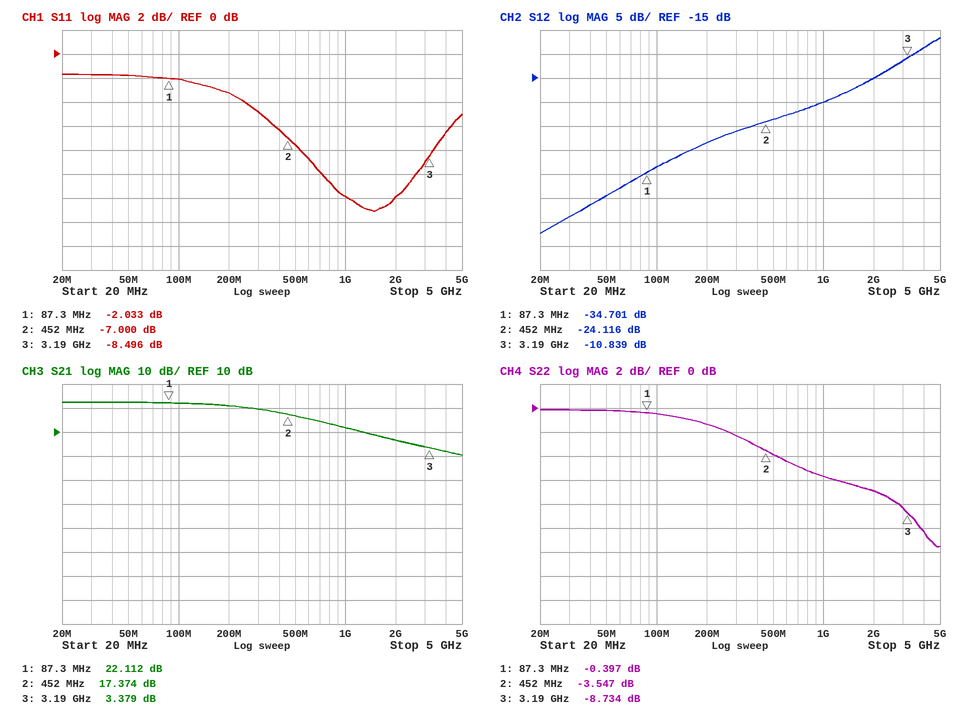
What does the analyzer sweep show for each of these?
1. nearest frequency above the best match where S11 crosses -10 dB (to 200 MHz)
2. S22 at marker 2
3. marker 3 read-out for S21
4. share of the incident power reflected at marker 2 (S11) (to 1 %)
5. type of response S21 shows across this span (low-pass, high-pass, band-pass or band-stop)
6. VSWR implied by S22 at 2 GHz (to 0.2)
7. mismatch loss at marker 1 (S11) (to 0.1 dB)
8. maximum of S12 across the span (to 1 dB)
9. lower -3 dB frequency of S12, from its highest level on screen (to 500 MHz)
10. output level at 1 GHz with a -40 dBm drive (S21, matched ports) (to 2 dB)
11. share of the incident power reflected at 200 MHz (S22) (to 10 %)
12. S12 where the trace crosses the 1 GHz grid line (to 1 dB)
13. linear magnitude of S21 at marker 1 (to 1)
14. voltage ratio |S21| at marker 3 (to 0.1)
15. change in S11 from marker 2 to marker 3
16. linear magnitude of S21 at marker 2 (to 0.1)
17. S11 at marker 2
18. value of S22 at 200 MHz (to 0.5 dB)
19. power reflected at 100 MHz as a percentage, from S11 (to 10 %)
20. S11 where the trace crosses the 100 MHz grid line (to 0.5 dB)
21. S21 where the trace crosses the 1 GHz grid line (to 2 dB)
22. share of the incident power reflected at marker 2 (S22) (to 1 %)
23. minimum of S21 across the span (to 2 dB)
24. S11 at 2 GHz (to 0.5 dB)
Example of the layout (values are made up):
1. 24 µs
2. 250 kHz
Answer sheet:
1. 2.6 GHz
2. -3.547 dB
3. 3.379 dB
4. 20 %
5. low-pass
6. 2.6
7. 4.3 dB
8. -7 dB
9. 3.5 GHz
10. -28 dBm
11. 70 %
12. -20 dB
13. 13
14. 1.5
15. -1.496 dB
16. 7.4
17. -7.000 dB
18. -1.5 dB
19. 60 %
20. -2.0 dB
21. 12 dB
22. 44 %
23. 0 dB
24. -12.0 dB
